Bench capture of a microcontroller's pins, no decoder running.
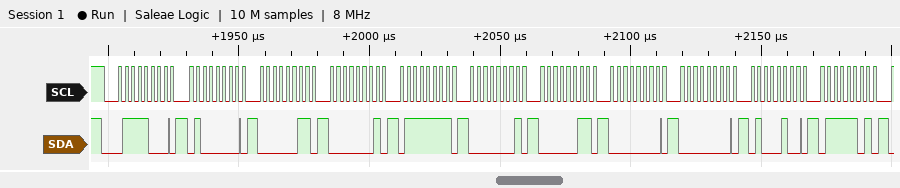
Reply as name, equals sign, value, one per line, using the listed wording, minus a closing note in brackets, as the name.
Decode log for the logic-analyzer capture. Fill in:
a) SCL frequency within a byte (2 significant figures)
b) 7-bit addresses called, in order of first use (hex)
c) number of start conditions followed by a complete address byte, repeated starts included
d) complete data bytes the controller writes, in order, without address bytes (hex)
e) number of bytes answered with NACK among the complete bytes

SCL frequency within a byte = 400 kHz
7-bit addresses called, in order of first use = 0x3C
number of start conditions followed by a complete address byte, repeated starts included = 1
complete data bytes the controller writes, in order, without address bytes = 40 03 01 7F 01 03 00 00 44 7D
number of bytes answered with NACK among the complete bytes = 0
